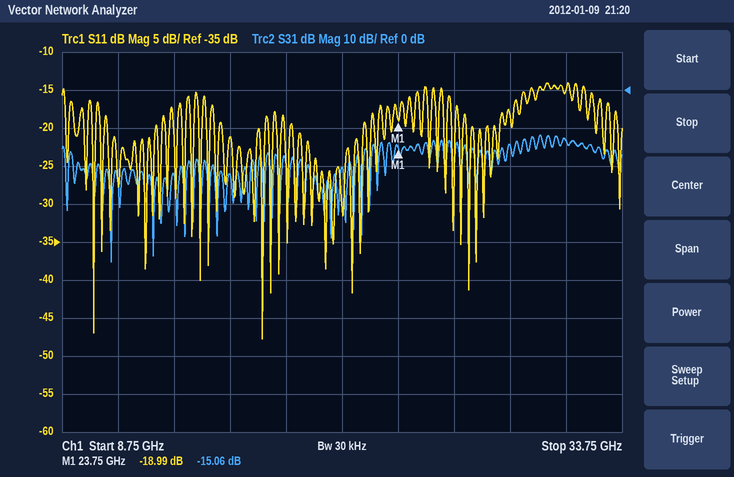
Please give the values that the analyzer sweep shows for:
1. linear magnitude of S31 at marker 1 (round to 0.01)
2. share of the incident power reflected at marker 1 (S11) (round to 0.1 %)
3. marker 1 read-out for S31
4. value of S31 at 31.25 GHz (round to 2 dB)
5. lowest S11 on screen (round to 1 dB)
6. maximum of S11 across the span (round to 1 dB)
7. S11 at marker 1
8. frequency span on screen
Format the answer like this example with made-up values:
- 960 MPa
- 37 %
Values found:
- 0.18
- 1.3 %
- -15.06 dB
- -14 dB
- -48 dB
- -14 dB
- -18.99 dB
- 25 GHz
